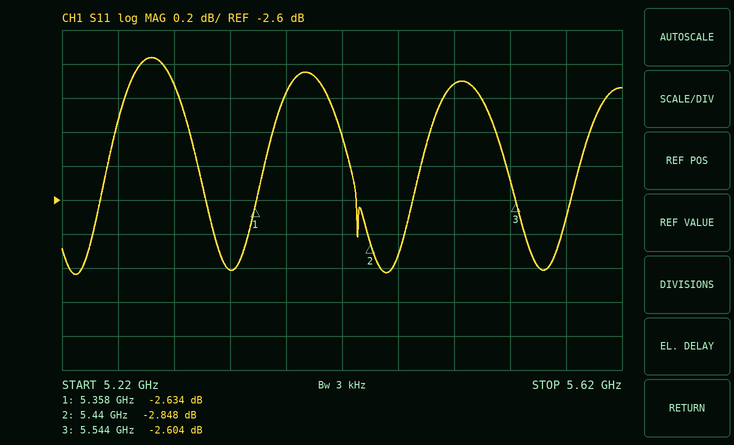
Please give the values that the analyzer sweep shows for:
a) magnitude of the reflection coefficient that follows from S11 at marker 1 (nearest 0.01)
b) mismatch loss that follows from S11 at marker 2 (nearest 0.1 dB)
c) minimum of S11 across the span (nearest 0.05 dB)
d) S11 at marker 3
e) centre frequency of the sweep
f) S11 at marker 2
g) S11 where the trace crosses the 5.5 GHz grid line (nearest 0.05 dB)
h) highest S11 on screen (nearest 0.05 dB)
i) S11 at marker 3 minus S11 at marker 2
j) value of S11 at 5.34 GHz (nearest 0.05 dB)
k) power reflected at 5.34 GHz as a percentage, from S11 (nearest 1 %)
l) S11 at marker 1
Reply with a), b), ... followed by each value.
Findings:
a) 0.74
b) 3.2 dB
c) -3.05 dB
d) -2.604 dB
e) 5.42 GHz
f) -2.848 dB
g) -1.90 dB
h) -1.75 dB
i) 0.244 dB
j) -3.00 dB
k) 50 %
l) -2.634 dB
